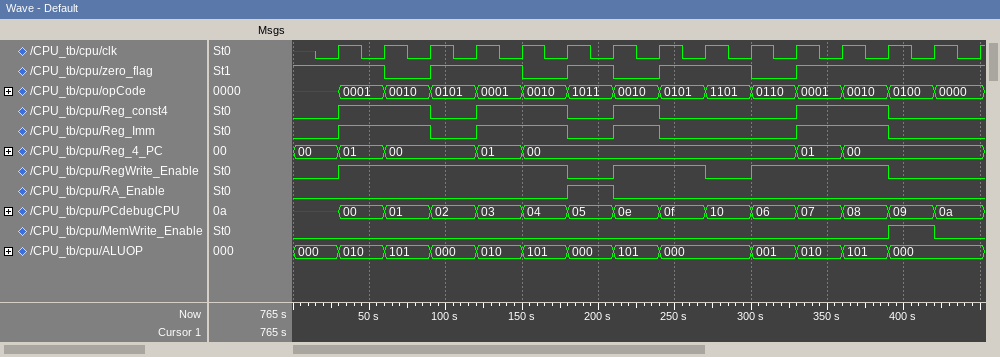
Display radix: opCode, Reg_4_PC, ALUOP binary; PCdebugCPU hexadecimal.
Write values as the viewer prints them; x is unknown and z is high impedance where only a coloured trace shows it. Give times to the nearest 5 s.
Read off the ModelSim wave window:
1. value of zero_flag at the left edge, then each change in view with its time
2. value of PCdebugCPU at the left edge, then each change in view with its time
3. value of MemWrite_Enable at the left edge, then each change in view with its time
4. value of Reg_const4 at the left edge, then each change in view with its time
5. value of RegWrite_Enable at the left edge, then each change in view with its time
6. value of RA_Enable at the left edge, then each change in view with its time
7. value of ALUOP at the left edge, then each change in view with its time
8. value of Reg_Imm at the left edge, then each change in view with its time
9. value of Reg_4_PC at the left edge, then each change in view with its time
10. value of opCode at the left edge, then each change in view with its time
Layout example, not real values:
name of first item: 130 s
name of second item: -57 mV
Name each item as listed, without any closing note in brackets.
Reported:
value of zero_flag at the left edge, then each change in view with its time: 1, 0 at 60 s, 1 at 90 s, 0 at 150 s, 1 at 180 s, 0 at 210 s, 1 at 240 s, 0 at 300 s, 1 at 330 s
value of PCdebugCPU at the left edge, then each change in view with its time: x, 00 at 30 s, 01 at 60 s, 02 at 90 s, 03 at 120 s, 04 at 150 s, 05 at 180 s, 0e at 210 s, 0f at 240 s, 10 at 270 s, 06 at 300 s, 07 at 330 s, 08 at 360 s, 09 at 390 s, 0a at 420 s
value of MemWrite_Enable at the left edge, then each change in view with its time: 0, 1 at 390 s, 0 at 420 s
value of Reg_const4 at the left edge, then each change in view with its time: 0, 1 at 30 s, 0 at 90 s, 1 at 120 s, 0 at 180 s, 1 at 210 s, 0 at 240 s, 1 at 330 s, 0 at 390 s
value of RegWrite_Enable at the left edge, then each change in view with its time: 0, 1 at 30 s, 0 at 180 s, 1 at 210 s, 0 at 270 s, 1 at 300 s, 0 at 390 s
value of RA_Enable at the left edge, then each change in view with its time: 0, 1 at 180 s, 0 at 210 s
value of ALUOP at the left edge, then each change in view with its time: 000, 010 at 30 s, 101 at 60 s, 000 at 90 s, 010 at 120 s, 101 at 150 s, 000 at 180 s, 101 at 210 s, 000 at 240 s, 001 at 300 s, 010 at 330 s, 101 at 360 s, 000 at 390 s
value of Reg_Imm at the left edge, then each change in view with its time: 0, 1 at 30 s, 0 at 90 s, 1 at 120 s, 0 at 180 s, 1 at 210 s, 0 at 240 s, 1 at 330 s, 0 at 390 s
value of Reg_4_PC at the left edge, then each change in view with its time: 00, 01 at 30 s, 00 at 60 s, 01 at 120 s, 00 at 150 s, 01 at 330 s, 00 at 360 s
value of opCode at the left edge, then each change in view with its time: x, 0001 at 30 s, 0010 at 60 s, 0101 at 90 s, 0001 at 120 s, 0010 at 150 s, 1011 at 180 s, 0010 at 210 s, 0101 at 240 s, 1101 at 270 s, 0110 at 300 s, 0001 at 330 s, 0010 at 360 s, 0100 at 390 s, 0000 at 420 s
